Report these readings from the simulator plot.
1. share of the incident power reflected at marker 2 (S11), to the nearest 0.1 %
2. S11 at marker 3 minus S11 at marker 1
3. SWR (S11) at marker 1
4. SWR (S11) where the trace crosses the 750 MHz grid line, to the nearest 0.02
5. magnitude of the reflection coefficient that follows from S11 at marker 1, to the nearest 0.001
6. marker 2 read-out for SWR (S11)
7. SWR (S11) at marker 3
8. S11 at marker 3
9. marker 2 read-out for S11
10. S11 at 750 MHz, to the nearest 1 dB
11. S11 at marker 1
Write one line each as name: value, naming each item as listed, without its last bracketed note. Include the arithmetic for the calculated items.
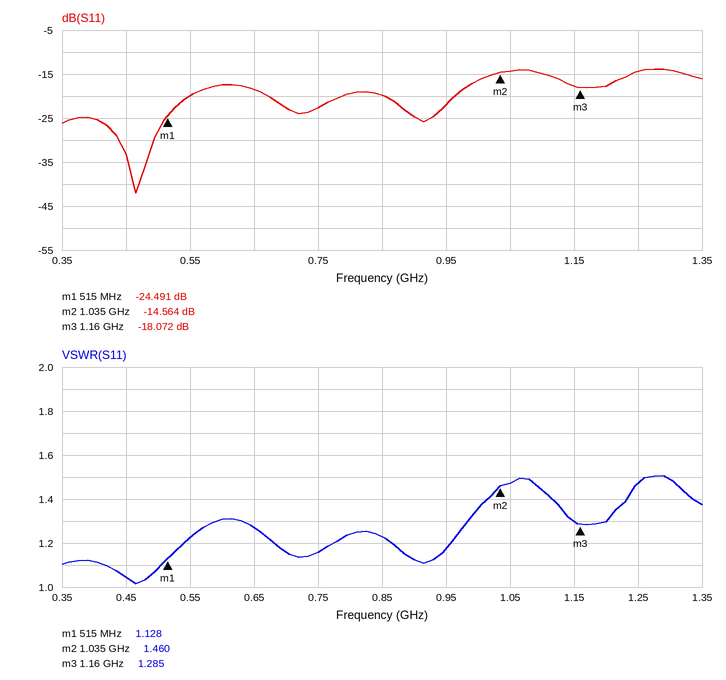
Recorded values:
share of the incident power reflected at marker 2 (S11), to the nearest 0.1 %: 10^(-14.564/10) ≈ 3.5 %
S11 at marker 3 minus S11 at marker 1: -18.072 − (-24.491) = 6.419 dB
SWR (S11) at marker 1: 1.128
SWR (S11) where the trace crosses the 750 MHz grid line, to the nearest 0.02: 1.16
magnitude of the reflection coefficient that follows from S11 at marker 1, to the nearest 0.001: 10^(-24.491/20) ≈ 0.060
marker 2 read-out for SWR: 1.460
SWR (S11) at marker 3: 1.285
S11 at marker 3: -18.072 dB
marker 2 read-out for S11: -14.564 dB
S11 at 750 MHz, to the nearest 1 dB: -23 dB
S11 at marker 1: -24.491 dB
